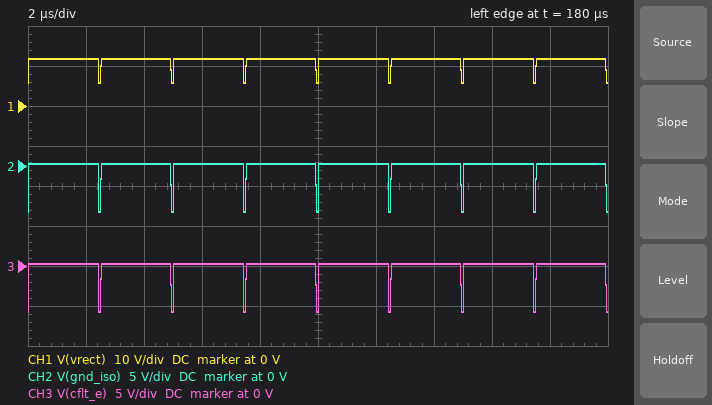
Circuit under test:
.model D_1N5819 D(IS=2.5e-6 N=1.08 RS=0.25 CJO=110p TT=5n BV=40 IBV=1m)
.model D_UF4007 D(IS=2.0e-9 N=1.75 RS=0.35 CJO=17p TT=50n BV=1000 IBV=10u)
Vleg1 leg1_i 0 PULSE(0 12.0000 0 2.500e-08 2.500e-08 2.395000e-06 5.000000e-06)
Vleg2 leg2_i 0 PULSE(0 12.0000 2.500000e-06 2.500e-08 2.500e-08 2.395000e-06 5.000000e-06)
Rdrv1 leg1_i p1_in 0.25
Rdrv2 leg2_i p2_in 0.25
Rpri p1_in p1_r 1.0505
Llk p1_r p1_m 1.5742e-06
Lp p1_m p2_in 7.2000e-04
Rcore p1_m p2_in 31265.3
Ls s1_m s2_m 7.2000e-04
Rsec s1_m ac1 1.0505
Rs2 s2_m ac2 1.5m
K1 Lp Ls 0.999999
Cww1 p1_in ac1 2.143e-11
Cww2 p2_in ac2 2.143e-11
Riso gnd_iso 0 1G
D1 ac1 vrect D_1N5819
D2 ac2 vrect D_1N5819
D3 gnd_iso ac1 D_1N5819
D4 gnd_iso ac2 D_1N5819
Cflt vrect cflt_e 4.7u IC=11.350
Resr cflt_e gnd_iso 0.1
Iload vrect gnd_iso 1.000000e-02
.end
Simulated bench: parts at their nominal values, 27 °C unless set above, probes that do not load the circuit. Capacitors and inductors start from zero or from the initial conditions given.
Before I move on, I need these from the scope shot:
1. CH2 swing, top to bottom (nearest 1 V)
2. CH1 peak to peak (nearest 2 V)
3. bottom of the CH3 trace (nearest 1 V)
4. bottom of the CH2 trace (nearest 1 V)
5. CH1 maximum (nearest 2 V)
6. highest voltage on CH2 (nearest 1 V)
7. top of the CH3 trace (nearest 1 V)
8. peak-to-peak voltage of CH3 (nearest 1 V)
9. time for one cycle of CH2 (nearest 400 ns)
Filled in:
6 V
6 V
-6 V
-6 V
12 V
0 V
0 V
6 V
2.4 µs
